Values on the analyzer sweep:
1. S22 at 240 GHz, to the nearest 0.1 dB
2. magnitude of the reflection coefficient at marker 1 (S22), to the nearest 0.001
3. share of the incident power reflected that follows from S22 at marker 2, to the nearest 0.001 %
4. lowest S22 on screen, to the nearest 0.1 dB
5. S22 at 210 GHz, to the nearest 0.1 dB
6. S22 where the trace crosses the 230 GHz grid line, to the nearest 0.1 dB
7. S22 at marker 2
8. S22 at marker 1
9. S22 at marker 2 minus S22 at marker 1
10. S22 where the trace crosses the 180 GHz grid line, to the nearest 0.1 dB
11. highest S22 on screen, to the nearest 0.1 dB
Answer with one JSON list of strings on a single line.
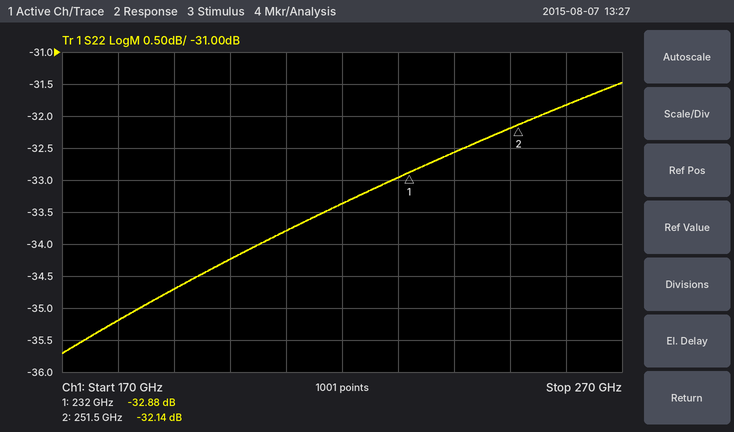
["-32.6 dB", "0.023", "0.061 %", "-35.7 dB", "-33.8 dB", "-33.0 dB", "-32.14 dB", "-32.88 dB", "0.74 dB", "-35.2 dB", "-31.5 dB"]
